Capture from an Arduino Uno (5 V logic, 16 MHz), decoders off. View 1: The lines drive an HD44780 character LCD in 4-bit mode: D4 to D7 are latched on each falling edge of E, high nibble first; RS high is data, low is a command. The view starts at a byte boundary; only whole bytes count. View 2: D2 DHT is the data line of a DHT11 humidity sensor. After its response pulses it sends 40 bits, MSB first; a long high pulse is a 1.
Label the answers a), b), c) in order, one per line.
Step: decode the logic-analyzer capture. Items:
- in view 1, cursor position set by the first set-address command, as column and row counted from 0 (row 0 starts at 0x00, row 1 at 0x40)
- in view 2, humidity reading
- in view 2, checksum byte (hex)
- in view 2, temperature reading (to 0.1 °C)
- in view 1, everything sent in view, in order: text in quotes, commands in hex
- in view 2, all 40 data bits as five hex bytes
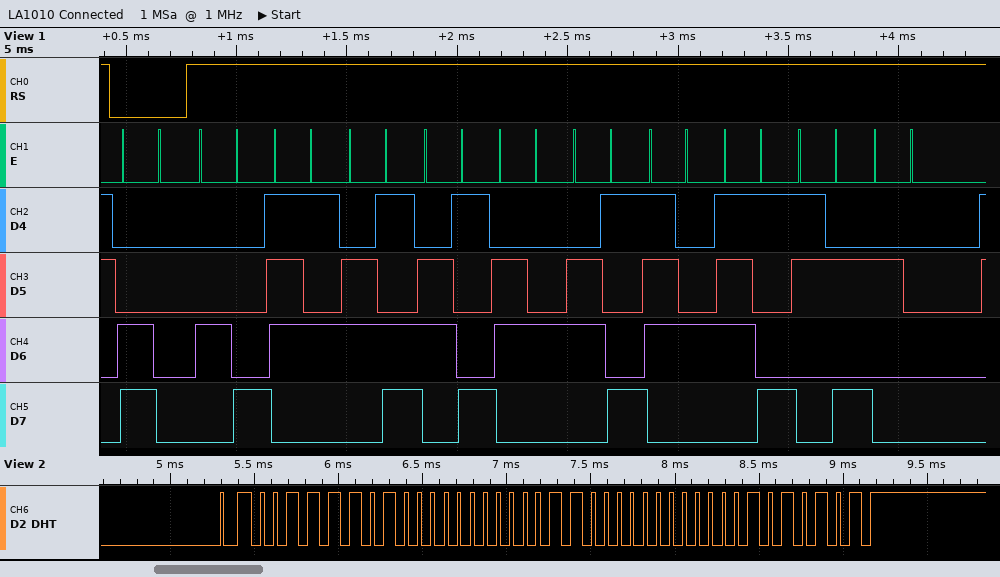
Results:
a) column 0, row 1
b) 61 %
c) 0x55
d) 24.0 °C
e) 0xC0 "Humidity: "
f) 3D 00 18 00 55
